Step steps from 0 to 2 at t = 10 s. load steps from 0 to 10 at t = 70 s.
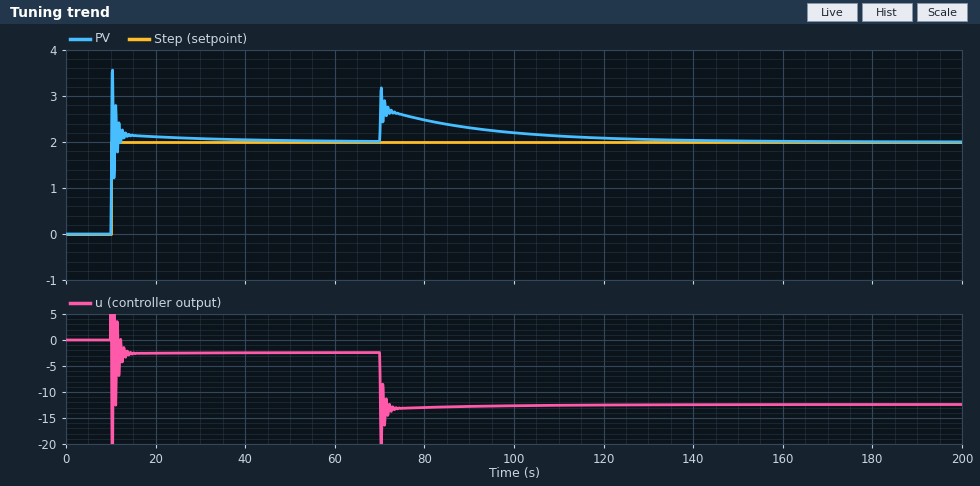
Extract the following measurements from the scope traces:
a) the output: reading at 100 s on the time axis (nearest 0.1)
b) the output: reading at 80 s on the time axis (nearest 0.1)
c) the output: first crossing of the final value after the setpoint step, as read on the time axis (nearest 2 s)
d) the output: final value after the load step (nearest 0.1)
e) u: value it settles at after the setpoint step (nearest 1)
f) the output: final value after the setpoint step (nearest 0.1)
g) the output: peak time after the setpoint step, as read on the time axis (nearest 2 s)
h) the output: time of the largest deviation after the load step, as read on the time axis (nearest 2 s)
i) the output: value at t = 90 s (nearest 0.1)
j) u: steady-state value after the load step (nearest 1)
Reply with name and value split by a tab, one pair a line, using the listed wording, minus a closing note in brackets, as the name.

the output: reading at 100 s on the time axis	2.2
the output: reading at 80 s on the time axis	2.5
the output: first crossing of the final value after the setpoint step, as read on the time axis	10 s
the output: final value after the load step	2.0
u: value it settles at after the setpoint step	-2
the output: final value after the setpoint step	2.0
the output: peak time after the setpoint step, as read on the time axis	10 s
the output: time of the largest deviation after the load step, as read on the time axis	70 s
the output: value at t = 90 s	2.3
u: steady-state value after the load step	-12
